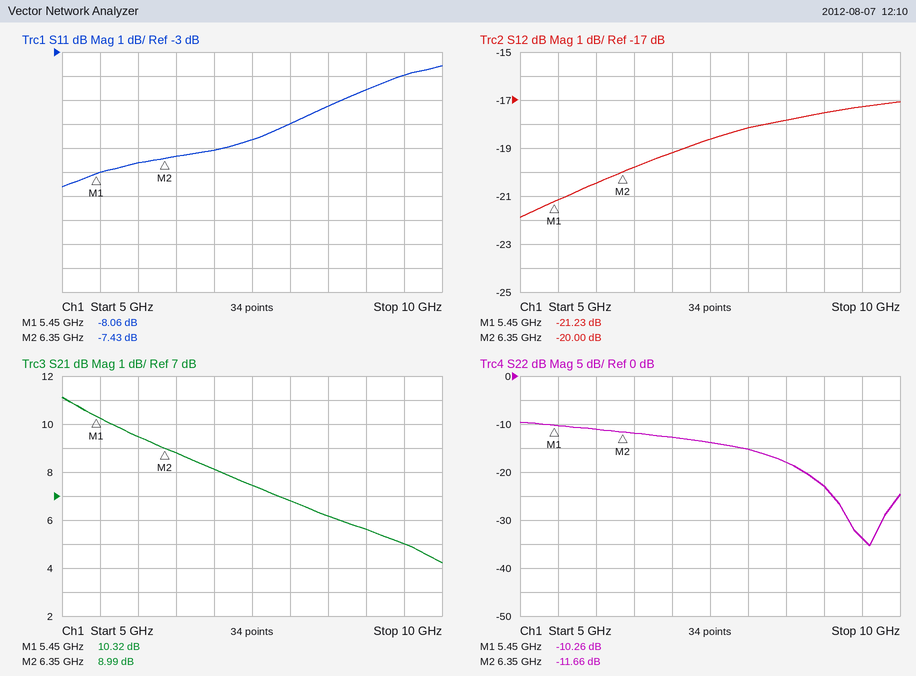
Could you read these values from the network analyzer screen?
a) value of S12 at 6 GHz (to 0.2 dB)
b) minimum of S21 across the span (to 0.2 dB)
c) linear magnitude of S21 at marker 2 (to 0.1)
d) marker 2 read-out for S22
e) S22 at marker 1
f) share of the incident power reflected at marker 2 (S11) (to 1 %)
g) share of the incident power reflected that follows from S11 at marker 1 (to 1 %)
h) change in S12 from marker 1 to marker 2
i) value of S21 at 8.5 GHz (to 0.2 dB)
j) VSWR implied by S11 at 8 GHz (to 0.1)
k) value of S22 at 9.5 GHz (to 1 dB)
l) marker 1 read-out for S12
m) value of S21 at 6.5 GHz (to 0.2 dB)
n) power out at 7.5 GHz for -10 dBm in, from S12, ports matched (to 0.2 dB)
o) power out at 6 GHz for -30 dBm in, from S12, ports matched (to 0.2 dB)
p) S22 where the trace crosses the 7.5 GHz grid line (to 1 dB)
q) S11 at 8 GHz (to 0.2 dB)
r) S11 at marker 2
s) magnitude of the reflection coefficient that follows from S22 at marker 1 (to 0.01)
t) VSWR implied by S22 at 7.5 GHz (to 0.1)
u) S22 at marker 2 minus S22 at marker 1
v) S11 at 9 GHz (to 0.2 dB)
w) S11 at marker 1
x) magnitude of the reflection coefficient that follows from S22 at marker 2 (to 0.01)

-20.4 dB
4.2 dB
2.8
-11.66 dB
-10.26 dB
18 %
16 %
1.23 dB
6.2 dB
3.0
-34 dB
-21.23 dB
8.8 dB
-28.6 dBm
-50.4 dBm
-14 dB
-6.0 dB
-7.43 dB
0.31
1.5
-1.40 dB
-4.6 dB
-8.06 dB
0.26
